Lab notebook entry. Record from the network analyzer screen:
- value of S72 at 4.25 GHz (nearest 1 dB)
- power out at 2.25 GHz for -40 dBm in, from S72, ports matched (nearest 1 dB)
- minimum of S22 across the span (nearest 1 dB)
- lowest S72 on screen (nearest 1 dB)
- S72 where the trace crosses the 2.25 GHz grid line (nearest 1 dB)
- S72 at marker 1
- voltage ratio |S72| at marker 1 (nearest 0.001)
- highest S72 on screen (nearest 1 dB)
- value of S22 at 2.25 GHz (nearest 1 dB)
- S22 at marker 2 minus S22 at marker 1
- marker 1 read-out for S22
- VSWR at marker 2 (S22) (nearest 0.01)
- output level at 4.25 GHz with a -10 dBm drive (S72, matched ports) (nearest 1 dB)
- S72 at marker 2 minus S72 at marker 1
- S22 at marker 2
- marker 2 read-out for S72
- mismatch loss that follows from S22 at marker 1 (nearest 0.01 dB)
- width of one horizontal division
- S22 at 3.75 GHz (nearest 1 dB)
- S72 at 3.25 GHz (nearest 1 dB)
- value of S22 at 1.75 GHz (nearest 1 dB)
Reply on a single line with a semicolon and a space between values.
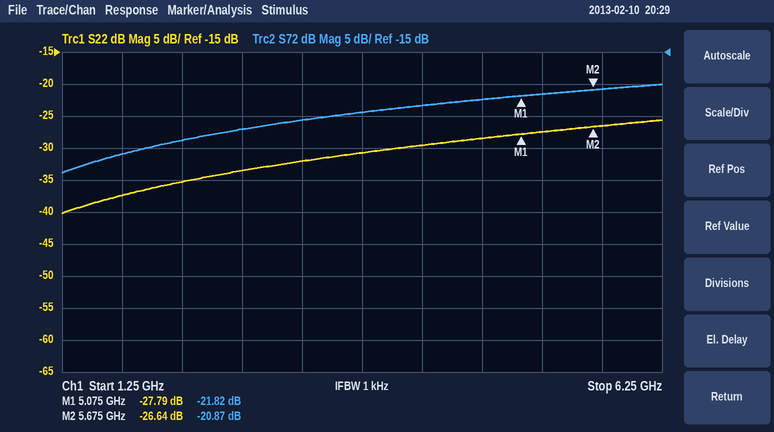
-23 dB; -69 dBm; -40 dB; -34 dB; -29 dB; -21.82 dB; 0.081; -20 dB; -35 dB; 1.15 dB; -27.79 dB; 1.10; -33 dBm; 0.95 dB; -26.64 dB; -20.87 dB; 0.01 dB; 500 MHz; -31 dB; -26 dB; -37 dB
